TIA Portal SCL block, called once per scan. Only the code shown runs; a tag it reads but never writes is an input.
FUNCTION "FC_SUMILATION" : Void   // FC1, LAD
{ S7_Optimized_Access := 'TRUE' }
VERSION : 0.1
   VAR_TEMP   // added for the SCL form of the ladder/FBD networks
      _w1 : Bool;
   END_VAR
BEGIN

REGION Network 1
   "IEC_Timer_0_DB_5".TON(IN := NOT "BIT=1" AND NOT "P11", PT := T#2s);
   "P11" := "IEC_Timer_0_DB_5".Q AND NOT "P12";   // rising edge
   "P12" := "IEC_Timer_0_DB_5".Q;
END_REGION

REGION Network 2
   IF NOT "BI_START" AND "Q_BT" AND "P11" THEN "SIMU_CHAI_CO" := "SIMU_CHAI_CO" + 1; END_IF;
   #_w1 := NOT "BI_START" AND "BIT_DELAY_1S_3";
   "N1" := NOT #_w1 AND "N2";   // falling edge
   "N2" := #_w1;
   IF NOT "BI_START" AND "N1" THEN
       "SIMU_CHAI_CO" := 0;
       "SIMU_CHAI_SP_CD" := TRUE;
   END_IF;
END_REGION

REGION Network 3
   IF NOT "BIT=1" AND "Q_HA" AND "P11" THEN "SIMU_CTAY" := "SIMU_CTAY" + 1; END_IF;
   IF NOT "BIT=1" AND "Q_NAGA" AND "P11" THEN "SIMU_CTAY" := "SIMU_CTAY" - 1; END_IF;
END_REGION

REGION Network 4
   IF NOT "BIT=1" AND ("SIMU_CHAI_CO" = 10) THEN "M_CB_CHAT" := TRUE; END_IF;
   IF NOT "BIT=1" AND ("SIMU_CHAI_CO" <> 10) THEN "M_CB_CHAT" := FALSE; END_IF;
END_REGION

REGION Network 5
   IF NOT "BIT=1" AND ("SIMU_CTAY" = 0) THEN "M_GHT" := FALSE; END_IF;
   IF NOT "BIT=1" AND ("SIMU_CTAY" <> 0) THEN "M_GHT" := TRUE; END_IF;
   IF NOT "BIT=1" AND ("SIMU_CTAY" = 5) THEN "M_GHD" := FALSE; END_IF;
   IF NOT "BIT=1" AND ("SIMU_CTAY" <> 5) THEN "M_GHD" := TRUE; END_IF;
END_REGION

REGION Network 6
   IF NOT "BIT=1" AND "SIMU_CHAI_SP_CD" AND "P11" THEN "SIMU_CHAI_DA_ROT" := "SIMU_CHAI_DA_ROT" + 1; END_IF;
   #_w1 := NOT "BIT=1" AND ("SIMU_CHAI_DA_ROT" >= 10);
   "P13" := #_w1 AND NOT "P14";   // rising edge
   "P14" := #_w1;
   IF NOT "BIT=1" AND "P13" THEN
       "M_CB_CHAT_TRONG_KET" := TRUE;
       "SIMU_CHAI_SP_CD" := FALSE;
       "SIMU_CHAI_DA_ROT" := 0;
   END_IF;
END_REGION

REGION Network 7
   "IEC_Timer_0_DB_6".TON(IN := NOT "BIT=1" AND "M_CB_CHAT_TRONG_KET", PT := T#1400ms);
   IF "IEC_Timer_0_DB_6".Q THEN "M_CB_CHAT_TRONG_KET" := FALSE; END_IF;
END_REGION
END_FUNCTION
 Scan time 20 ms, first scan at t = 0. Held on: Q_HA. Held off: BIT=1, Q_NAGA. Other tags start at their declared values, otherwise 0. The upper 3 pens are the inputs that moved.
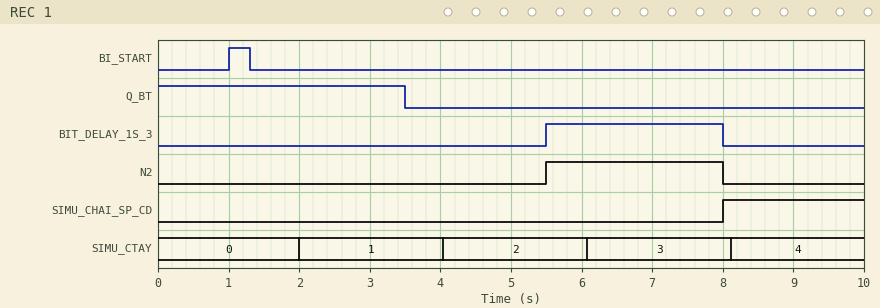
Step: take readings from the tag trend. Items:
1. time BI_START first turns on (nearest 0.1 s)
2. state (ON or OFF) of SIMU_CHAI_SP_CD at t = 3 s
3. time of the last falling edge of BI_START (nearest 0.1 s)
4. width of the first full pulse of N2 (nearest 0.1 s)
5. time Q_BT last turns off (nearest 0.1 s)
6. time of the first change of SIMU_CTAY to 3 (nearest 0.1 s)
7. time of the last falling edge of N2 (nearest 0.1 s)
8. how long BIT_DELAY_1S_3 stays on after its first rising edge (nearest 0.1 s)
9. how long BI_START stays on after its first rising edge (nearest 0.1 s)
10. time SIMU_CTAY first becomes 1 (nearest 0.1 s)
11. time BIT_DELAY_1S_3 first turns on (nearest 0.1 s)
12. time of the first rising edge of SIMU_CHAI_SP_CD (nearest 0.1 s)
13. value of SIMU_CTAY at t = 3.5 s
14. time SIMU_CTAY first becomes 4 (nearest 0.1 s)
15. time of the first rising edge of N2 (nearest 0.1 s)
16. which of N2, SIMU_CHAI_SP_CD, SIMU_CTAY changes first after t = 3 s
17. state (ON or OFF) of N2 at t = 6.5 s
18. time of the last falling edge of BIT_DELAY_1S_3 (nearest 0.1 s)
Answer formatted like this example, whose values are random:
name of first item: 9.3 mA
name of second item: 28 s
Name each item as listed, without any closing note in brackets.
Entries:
time BI_START first turns on: 1.0 s
state (ON or OFF) of SIMU_CHAI_SP_CD at t = 3 s: OFF
time of the last falling edge of BI_START: 1.3 s
width of the first full pulse of N2: 2.5 s
time Q_BT last turns off: 3.5 s
time of the first change of SIMU_CTAY to 3: 6.1 s
time of the last falling edge of N2: 8.0 s
how long BIT_DELAY_1S_3 stays on after its first rising edge: 2.5 s
how long BI_START stays on after its first rising edge: 0.3 s
time SIMU_CTAY first becomes 1: 2.0 s
time BIT_DELAY_1S_3 first turns on: 5.5 s
time of the first rising edge of SIMU_CHAI_SP_CD: 8.0 s
value of SIMU_CTAY at t = 3.5 s: 1
time SIMU_CTAY first becomes 4: 8.1 s
time of the first rising edge of N2: 5.5 s
which of N2, SIMU_CHAI_SP_CD, SIMU_CTAY changes first after t = 3 s: SIMU_CTAY
state (ON or OFF) of N2 at t = 6.5 s: ON
time of the last falling edge of BIT_DELAY_1S_3: 8.0 s
